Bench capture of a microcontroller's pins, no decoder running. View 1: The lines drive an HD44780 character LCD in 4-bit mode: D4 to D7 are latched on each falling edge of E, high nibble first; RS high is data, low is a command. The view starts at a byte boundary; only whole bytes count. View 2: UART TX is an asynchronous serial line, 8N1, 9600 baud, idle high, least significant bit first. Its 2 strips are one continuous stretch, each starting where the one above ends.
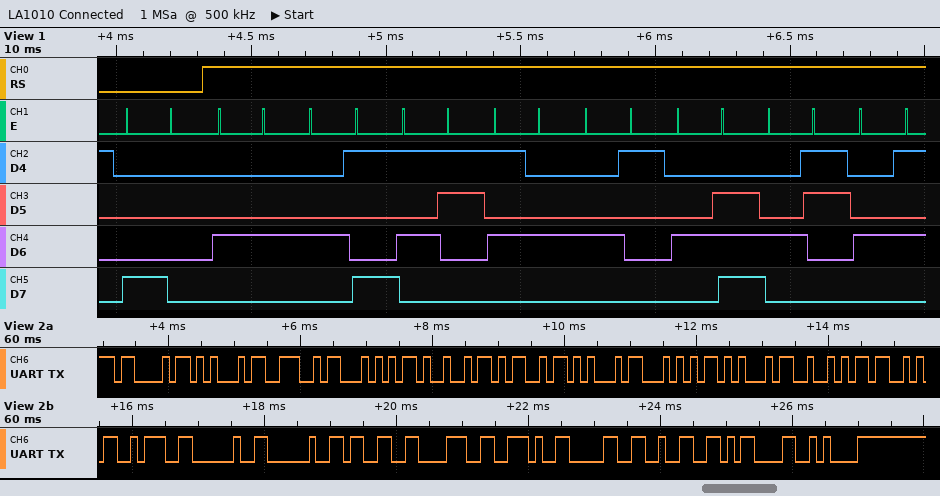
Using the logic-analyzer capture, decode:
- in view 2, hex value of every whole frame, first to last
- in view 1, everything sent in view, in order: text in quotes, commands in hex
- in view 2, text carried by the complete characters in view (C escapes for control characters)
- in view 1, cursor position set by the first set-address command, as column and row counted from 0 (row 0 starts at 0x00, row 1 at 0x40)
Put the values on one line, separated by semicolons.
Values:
43 45 4E 54 49 4D 45 54 45 52 53 3A 20 20 33 38 2E 30 32 0D 0A; 0x80 "DISTANCE"; "CENTIMETERS:  38.02\r\n"; column 0, row 0
